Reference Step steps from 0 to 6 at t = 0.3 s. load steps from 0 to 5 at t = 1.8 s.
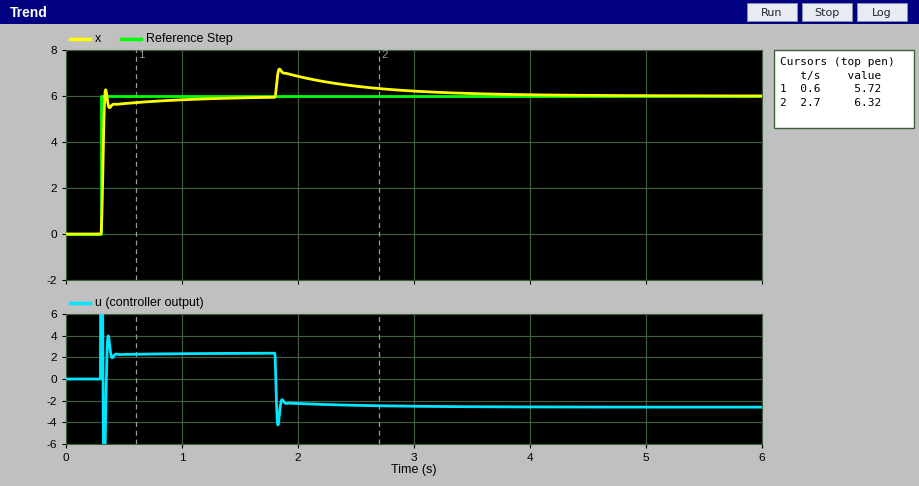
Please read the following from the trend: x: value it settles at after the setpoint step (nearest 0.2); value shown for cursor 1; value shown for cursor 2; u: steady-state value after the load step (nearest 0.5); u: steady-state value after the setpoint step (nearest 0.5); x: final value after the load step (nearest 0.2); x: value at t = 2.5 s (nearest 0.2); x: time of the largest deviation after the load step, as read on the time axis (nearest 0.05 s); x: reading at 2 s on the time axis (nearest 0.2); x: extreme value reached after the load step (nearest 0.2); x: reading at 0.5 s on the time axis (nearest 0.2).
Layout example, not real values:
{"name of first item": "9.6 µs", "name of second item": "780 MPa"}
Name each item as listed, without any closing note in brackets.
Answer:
{"x: value it settles at after the setpoint step": "6.0", "value shown for cursor 1": "5.72", "value shown for cursor 2": "6.32", "u: steady-state value after the load step": "-2.5", "u: steady-state value after the setpoint step": "2.5", "x: final value after the load step": "6.0", "x: value at t = 2.5 s": "6.4", "x: time of the largest deviation after the load step, as read on the time axis": "1.85 s", "x: reading at 2 s on the time axis": "6.8", "x: extreme value reached after the load step": "7.2", "x: reading at 0.5 s on the time axis": "5.6"}
